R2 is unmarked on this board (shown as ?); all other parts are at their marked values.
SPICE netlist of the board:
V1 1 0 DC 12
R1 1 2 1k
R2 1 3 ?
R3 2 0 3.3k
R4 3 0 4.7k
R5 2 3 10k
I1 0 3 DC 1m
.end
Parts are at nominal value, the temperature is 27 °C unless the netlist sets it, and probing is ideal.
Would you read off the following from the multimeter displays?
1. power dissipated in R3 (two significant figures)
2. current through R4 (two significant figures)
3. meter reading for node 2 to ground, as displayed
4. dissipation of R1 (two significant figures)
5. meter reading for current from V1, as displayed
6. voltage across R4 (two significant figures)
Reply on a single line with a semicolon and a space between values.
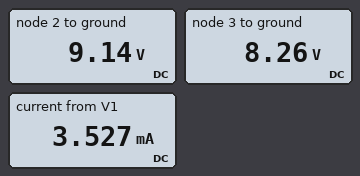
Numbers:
25 mW; 1.8 mA; 9.14 V; 8.2 mW; 3.527 mA; 8.3 V
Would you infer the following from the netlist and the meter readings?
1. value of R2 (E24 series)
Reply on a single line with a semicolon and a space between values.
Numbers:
5.6 kΩ
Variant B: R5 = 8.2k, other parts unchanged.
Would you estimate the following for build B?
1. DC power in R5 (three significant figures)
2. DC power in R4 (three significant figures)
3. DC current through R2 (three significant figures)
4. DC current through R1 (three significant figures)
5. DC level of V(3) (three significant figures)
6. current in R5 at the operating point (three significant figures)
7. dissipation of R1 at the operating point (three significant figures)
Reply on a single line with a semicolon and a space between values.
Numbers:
85.7 µW; 14.6 mW; 662 µA; 2.87 mA; 8.29 V; 102 µA; 8.23 mW
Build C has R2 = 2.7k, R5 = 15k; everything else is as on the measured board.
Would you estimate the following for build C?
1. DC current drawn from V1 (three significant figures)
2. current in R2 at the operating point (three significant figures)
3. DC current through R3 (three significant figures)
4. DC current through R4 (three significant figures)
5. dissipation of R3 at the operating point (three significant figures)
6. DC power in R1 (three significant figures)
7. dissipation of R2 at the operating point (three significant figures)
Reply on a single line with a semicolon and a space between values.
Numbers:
3.78 mA; 991 µA; 2.79 mA; 1.98 mA; 25.7 mW; 7.76 mW; 2.65 mW
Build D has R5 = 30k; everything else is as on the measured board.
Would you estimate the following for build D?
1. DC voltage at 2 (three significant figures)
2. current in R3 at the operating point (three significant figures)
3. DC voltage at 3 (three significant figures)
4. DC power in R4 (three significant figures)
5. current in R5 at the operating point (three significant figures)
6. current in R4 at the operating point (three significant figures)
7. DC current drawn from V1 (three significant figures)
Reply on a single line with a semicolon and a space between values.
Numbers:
9.18 V; 2.78 mA; 8.12 V; 14.0 mW; 35.4 µA; 1.73 mA; 3.51 mA
